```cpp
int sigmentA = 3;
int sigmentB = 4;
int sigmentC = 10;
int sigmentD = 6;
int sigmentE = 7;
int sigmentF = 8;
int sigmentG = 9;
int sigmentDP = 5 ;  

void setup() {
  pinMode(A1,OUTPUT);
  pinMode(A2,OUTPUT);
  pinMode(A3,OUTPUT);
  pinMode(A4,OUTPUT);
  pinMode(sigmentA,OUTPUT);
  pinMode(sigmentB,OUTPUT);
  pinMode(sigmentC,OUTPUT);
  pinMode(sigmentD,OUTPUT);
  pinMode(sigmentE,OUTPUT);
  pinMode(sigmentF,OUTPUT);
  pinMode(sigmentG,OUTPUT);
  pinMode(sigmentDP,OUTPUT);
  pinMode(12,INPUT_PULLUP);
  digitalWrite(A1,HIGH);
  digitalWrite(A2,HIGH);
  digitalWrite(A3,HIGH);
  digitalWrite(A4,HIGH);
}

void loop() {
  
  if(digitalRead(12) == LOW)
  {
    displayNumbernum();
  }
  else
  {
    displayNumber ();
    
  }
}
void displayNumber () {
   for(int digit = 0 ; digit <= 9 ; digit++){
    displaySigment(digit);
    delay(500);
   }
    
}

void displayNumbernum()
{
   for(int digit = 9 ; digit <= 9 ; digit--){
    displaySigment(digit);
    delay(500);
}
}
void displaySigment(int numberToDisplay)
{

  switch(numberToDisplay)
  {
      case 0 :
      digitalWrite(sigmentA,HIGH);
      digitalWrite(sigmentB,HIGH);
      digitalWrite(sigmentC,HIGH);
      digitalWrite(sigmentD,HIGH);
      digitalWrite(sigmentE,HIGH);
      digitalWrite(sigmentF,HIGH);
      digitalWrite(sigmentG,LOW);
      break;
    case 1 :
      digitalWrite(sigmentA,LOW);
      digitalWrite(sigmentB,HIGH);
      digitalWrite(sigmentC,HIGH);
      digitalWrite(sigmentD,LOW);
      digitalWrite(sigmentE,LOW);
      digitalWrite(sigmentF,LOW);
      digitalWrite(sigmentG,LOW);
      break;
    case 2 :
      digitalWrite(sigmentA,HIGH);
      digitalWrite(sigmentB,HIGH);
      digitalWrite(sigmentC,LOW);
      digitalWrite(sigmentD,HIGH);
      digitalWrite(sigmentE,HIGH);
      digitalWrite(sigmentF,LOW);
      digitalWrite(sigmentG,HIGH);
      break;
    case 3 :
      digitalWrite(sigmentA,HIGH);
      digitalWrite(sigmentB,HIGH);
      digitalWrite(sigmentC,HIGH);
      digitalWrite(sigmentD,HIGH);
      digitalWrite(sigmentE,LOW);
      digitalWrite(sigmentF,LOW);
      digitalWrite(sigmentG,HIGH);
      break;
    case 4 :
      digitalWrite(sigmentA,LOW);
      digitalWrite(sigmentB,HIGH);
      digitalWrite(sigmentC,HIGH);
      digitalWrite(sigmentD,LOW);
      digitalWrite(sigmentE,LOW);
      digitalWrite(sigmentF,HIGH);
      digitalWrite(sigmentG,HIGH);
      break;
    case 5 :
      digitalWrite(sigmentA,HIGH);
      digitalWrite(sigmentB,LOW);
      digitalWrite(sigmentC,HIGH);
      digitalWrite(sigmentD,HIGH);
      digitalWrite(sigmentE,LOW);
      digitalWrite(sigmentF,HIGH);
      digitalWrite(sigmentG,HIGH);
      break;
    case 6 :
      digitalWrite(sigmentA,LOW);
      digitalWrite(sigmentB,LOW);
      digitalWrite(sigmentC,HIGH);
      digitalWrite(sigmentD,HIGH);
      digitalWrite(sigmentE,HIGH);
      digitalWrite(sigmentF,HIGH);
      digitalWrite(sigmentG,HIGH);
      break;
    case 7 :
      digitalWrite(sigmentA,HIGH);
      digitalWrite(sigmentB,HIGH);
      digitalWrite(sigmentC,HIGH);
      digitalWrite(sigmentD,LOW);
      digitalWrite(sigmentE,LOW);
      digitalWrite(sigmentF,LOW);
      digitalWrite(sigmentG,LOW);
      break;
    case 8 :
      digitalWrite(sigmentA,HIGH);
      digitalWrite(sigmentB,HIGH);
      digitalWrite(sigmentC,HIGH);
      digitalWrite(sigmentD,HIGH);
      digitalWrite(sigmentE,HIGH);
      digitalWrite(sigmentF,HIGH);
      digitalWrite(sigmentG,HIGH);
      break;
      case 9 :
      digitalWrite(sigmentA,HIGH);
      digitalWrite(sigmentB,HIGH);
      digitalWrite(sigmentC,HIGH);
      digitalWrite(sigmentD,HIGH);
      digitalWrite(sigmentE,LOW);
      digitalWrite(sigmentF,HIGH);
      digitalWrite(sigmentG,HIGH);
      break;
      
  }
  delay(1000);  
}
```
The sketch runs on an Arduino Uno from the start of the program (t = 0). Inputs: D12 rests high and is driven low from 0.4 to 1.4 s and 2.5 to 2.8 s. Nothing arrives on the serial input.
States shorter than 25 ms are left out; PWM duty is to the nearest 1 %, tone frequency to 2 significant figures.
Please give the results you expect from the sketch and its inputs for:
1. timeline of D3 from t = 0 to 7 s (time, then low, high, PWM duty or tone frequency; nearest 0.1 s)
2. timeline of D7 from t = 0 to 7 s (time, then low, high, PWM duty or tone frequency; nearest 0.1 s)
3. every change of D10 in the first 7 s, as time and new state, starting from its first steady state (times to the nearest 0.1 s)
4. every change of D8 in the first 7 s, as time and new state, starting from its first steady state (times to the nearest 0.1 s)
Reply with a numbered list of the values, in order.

1. 0 s high; 1.5 s low; 3 s high; 6 s low
2. 0 s high; 1.5 s low; 3 s high; 4.5 s low
3. 0 s high; 3 s low; 4.5 s high
4. 0 s high; 1.5 s low; 6 s high
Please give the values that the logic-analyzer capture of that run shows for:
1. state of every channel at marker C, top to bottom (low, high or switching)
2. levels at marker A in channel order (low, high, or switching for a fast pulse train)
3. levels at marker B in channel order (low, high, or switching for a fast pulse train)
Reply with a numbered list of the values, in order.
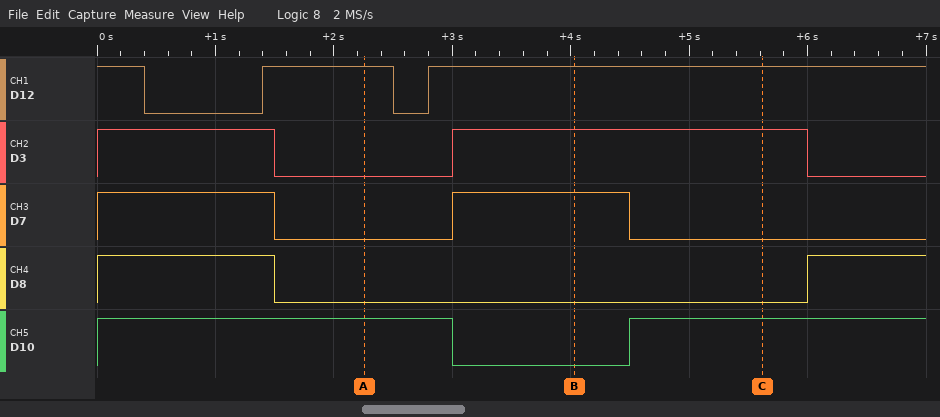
1. D12 high, D3 high, D7 low, D8 low, D10 high
2. D12 high, D3 low, D7 low, D8 low, D10 high
3. D12 high, D3 high, D7 high, D8 low, D10 low
